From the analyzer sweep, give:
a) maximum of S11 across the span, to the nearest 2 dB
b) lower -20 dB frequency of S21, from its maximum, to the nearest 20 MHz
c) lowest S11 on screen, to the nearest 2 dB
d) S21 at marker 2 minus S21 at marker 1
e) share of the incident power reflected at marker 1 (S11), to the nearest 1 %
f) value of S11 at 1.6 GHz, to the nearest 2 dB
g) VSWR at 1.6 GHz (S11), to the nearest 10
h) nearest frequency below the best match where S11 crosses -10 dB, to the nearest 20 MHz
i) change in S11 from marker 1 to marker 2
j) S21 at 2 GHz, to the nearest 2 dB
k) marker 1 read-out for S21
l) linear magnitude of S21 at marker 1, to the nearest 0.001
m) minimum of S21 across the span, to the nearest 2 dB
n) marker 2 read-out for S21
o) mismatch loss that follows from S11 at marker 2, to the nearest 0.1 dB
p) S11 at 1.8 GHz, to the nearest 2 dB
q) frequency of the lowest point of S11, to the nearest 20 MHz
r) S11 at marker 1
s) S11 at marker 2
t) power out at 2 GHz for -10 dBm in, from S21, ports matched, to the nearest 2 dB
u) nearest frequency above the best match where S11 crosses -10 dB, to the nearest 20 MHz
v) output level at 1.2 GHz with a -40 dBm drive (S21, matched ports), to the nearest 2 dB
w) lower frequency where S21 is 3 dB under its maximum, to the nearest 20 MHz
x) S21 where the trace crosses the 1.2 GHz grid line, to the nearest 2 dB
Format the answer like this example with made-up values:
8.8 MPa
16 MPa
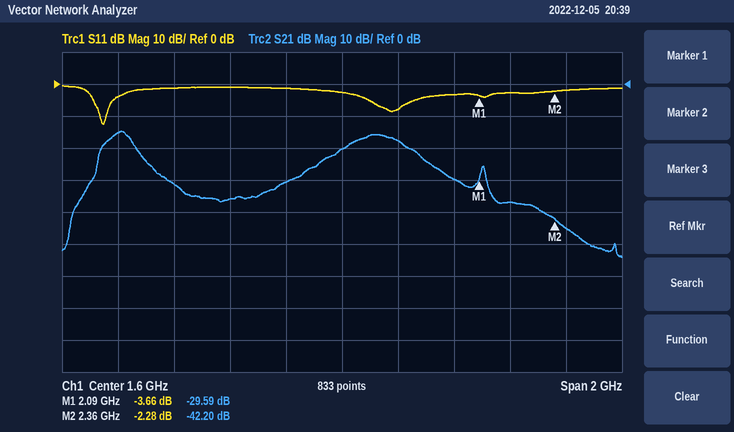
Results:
0 dB
680 MHz
-12 dB
-12.61 dB
43 %
-2 dB
10
740 MHz
1.38 dB
-30 dB
-29.59 dB
0.033
-54 dB
-42.20 dB
3.9 dB
-8 dB
740 MHz
-3.66 dB
-2.28 dB
-40 dBm
760 MHz
-76 dBm
760 MHz
-36 dB
